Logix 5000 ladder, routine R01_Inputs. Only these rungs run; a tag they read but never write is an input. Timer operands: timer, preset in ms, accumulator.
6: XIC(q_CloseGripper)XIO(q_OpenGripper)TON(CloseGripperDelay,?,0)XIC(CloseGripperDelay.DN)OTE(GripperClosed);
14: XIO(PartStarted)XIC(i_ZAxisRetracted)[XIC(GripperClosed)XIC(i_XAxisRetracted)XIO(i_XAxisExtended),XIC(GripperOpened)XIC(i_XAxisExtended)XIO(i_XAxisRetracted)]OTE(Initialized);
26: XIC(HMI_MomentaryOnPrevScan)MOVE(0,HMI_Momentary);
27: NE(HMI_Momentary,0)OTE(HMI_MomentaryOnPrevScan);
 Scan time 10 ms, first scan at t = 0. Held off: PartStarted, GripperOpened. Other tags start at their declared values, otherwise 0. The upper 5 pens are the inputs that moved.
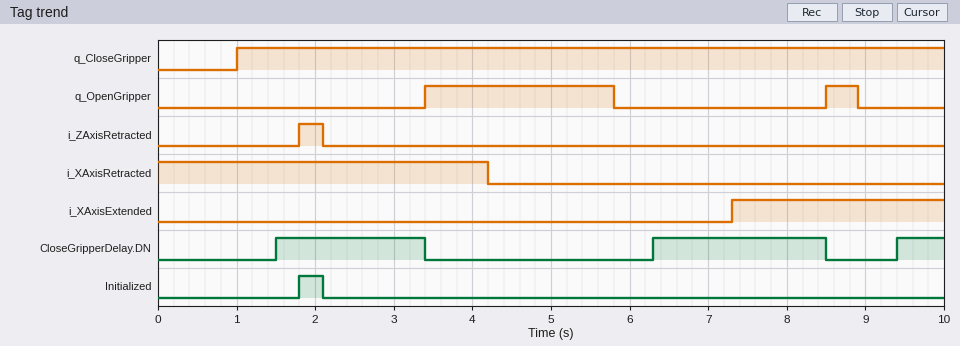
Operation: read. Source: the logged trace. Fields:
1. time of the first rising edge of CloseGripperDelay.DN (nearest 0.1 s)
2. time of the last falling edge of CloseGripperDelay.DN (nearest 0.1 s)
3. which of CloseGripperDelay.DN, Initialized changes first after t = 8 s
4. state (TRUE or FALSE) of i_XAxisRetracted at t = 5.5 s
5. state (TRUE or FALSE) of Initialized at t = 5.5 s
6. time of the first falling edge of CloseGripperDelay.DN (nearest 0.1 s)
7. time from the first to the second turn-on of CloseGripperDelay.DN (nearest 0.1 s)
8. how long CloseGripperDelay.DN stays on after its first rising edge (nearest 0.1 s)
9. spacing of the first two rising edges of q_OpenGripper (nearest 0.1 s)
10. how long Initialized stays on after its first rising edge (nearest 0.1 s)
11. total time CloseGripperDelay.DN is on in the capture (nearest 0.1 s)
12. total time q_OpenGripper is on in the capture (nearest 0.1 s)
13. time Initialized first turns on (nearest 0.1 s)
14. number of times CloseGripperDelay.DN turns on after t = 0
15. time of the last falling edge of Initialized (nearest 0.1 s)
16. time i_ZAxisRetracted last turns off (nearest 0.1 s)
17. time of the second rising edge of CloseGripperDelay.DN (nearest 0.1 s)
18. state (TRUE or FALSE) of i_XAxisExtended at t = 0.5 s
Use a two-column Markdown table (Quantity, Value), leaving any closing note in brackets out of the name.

| Quantity | Value |
|---|---|
| time of the first rising edge of CloseGripperDelay.DN | 1.5 s |
| time of the last falling edge of CloseGripperDelay.DN | 8.5 s |
| which of CloseGripperDelay.DN, Initialized changes first after t = 8 s | CloseGripperDelay.DN |
| state (TRUE or FALSE) of i_XAxisRetracted at t = 5.5 s | FALSE |
| state (TRUE or FALSE) of Initialized at t = 5.5 s | FALSE |
| time of the first falling edge of CloseGripperDelay.DN | 3.4 s |
| time from the first to the second turn-on of CloseGripperDelay.DN | 4.8 s |
| how long CloseGripperDelay.DN stays on after its first rising edge | 1.9 s |
| spacing of the first two rising edges of q_OpenGripper | 5.1 s |
| how long Initialized stays on after its first rising edge | 0.3 s |
| total time CloseGripperDelay.DN is on in the capture | 4.7 s |
| total time q_OpenGripper is on in the capture | 2.8 s |
| time Initialized first turns on | 1.8 s |
| number of times CloseGripperDelay.DN turns on after t = 0 | 3 |
| time of the last falling edge of Initialized | 2.1 s |
| time i_ZAxisRetracted last turns off | 2.1 s |
| time of the second rising edge of CloseGripperDelay.DN | 6.3 s |
| state (TRUE or FALSE) of i_XAxisExtended at t = 0.5 s | FALSE |
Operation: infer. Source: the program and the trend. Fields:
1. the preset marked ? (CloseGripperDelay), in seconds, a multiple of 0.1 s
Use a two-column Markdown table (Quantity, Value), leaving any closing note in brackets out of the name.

| Quantity | Value |
|---|---|
| the preset marked ? (CloseGripperDelay), in seconds, a multiple of 0.1 s | 0.5 s |
